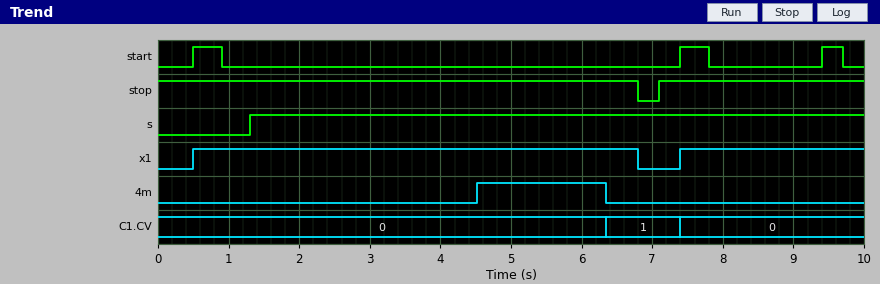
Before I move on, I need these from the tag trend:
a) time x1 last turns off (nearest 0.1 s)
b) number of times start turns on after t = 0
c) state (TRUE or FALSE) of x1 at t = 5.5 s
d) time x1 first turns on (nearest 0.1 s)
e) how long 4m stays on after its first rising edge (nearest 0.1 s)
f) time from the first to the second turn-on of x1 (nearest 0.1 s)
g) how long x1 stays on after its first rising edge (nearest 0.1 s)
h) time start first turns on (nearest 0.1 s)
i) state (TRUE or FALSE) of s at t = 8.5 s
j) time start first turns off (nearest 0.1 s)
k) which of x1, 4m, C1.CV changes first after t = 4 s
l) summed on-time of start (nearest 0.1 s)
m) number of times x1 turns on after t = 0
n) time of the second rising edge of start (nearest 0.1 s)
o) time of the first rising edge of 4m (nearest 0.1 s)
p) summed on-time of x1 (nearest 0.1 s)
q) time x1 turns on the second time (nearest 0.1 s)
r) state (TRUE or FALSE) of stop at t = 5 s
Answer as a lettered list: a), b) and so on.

a) 6.8 s
b) 3
c) TRUE
d) 0.5 s
e) 1.8 s
f) 6.9 s
g) 6.3 s
h) 0.5 s
i) TRUE
j) 0.9 s
k) 4m
l) 1.1 s
m) 2
n) 7.4 s
o) 4.5 s
p) 8.9 s
q) 7.4 s
r) TRUE
